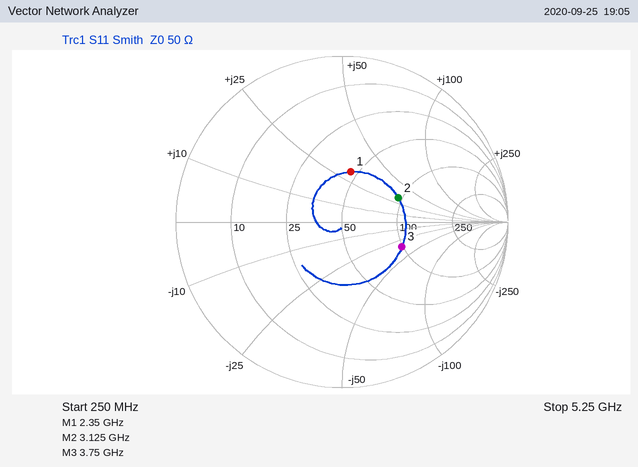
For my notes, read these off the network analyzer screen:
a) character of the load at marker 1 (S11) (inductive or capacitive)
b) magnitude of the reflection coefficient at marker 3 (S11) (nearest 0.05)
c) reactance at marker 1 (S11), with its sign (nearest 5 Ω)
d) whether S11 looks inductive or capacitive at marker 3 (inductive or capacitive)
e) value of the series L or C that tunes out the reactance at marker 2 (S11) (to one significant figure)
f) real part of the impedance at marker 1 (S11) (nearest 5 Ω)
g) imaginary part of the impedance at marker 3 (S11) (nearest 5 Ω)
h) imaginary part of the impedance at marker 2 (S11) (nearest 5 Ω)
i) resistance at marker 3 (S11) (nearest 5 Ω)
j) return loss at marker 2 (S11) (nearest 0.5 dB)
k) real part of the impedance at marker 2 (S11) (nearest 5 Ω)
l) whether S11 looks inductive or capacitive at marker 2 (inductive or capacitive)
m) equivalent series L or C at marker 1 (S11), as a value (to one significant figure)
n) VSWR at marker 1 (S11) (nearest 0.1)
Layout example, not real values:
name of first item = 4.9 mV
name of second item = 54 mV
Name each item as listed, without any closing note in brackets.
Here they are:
character of the load at marker 1 (S11) = inductive
magnitude of the reflection coefficient at marker 3 (S11) = 0.40
reactance at marker 1 (S11), with its sign = +30 Ω
whether S11 looks inductive or capacitive at marker 3 = capacitive
value of the series L or C that tunes out the reactance at marker 2 (S11) = 2 pF
real part of the impedance at marker 1 (S11) = 45 Ω
imaginary part of the impedance at marker 3 (S11) = -35 Ω
imaginary part of the impedance at marker 2 (S11) = +30 Ω
resistance at marker 3 (S11) = 100 Ω
return loss at marker 2 (S11) = 8.5 dB
real part of the impedance at marker 2 (S11) = 95 Ω
whether S11 looks inductive or capacitive at marker 2 = inductive
equivalent series L or C at marker 1 (S11), as a value = 2 nH
VSWR at marker 1 (S11) = 1.9
